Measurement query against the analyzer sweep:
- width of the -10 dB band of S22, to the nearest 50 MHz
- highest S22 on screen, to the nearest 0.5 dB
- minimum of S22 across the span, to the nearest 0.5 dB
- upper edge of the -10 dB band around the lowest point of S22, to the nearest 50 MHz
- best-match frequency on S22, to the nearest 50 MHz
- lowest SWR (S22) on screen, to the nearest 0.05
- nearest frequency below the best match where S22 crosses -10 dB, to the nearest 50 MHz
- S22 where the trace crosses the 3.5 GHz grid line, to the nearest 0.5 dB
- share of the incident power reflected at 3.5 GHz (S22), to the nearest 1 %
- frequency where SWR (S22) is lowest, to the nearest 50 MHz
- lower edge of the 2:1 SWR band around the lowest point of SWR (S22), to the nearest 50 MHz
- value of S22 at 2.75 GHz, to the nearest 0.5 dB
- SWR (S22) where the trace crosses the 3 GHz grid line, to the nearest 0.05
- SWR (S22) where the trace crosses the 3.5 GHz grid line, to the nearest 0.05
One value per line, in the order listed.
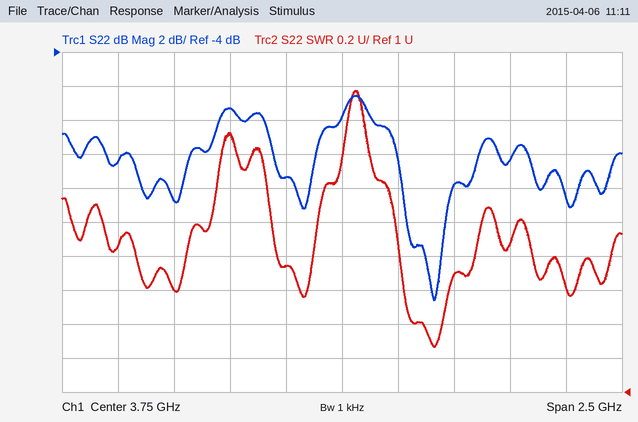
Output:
350 MHz
-6.5 dB
-18.5 dB
4.35 GHz
4.15 GHz
1.25
4.00 GHz
-11.5 dB
7 %
4.15 GHz
4.00 GHz
-10.5 dB
1.60
1.75
